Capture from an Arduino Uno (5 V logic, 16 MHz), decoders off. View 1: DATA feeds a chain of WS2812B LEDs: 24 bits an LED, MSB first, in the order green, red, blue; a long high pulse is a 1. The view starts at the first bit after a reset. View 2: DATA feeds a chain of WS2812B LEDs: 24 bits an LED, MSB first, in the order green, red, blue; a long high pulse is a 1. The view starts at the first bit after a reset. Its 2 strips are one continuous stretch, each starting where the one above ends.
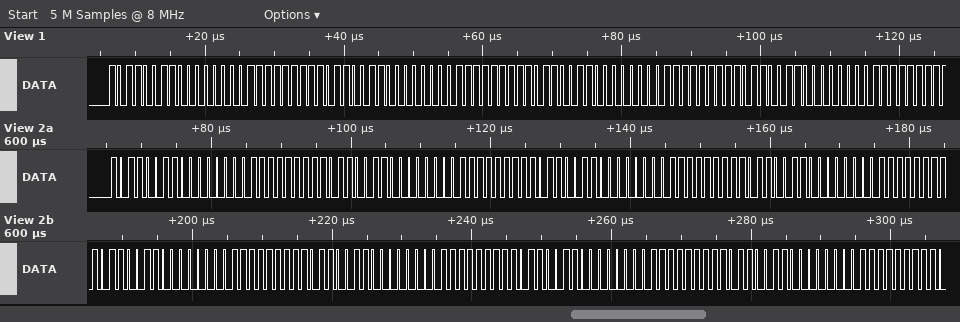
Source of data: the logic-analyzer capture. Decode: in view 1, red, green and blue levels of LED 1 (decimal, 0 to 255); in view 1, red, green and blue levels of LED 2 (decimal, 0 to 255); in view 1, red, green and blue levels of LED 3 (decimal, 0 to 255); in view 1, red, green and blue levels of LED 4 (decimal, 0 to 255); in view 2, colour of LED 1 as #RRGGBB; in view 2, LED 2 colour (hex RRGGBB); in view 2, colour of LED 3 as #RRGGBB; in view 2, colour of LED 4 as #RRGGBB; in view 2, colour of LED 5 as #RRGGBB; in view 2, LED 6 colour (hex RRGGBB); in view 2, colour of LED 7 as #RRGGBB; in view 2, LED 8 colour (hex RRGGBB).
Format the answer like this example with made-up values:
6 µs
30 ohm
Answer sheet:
0, 179, 255
0, 179, 255
0, 179, 255
0, 179, 255
#00B3FF
#00B3FF
#00B3FF
#00B3FF
#00B3FF
#00B3FF
#00B3FF
#00B3FF
